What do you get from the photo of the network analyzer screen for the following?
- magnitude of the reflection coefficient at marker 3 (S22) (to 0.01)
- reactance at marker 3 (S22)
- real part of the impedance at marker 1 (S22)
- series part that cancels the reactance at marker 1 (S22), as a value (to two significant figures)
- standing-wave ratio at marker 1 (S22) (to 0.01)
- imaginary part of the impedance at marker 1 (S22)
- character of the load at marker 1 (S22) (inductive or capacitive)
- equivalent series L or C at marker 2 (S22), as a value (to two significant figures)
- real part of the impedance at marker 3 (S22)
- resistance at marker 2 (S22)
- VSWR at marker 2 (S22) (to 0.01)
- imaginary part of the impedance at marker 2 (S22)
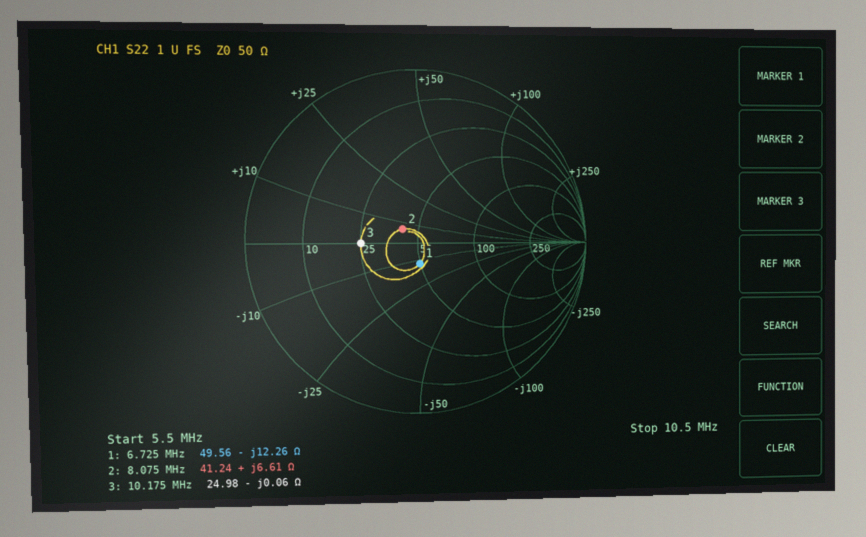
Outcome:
0.33
-0.06 Ω
49.56 Ω
290 nH
1.28
-12.26 Ω
capacitive
130 nH
24.98 Ω
41.24 Ω
1.27
+6.61 Ω
